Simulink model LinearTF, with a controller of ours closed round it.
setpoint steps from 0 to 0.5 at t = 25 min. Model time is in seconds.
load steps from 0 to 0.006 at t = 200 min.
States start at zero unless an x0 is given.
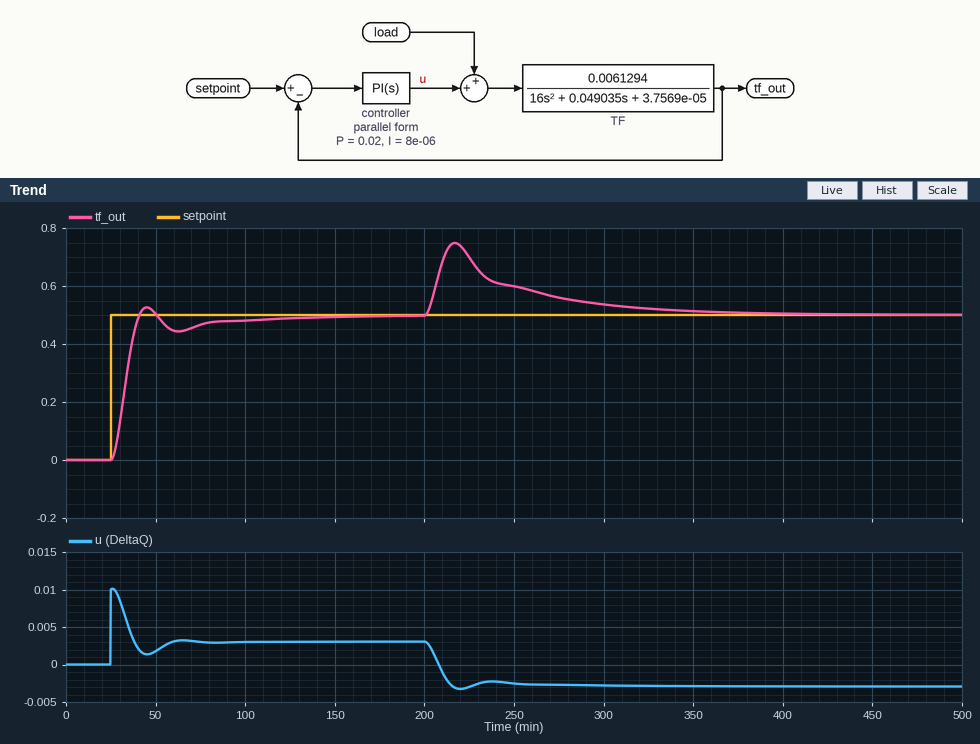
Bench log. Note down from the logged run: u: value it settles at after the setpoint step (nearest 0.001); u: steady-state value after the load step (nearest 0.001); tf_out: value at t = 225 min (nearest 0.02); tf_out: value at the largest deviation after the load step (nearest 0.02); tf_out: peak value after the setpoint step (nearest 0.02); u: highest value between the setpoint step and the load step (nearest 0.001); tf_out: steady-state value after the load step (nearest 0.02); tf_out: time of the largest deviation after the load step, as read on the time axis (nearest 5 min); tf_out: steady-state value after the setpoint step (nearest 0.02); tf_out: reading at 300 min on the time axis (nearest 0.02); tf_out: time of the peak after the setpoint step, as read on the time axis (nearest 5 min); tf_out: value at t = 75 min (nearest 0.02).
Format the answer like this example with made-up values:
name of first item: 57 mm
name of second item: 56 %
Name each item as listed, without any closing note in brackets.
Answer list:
u: value it settles at after the setpoint step: 0.003
u: steady-state value after the load step: -0.003
tf_out: value at t = 225 min: 0.70
tf_out: value at the largest deviation after the load step: 0.74
tf_out: peak value after the setpoint step: 0.52
u: highest value between the setpoint step and the load step: 0.010
tf_out: steady-state value after the load step: 0.50
tf_out: time of the largest deviation after the load step, as read on the time axis: 215 min
tf_out: steady-state value after the setpoint step: 0.50
tf_out: reading at 300 min on the time axis: 0.54
tf_out: time of the peak after the setpoint step, as read on the time axis: 45 min
tf_out: value at t = 75 min: 0.46
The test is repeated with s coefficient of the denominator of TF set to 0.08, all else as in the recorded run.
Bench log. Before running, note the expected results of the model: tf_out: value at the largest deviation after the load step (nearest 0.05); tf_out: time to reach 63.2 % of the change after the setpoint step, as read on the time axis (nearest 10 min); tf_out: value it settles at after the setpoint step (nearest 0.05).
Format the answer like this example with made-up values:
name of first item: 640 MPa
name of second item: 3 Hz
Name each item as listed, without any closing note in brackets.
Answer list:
tf_out: value at the largest deviation after the load step: 0.70
tf_out: time to reach 63.2 % of the change after the setpoint step, as read on the time axis: 40 min
tf_out: value it settles at after the setpoint step: 0.50
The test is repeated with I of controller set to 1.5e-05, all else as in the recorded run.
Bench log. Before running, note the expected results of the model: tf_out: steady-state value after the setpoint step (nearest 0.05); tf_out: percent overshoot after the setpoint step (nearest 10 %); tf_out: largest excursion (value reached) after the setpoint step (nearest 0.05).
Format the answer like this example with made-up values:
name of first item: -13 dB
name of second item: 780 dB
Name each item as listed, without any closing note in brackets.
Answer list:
tf_out: steady-state value after the setpoint step: 0.50
tf_out: percent overshoot after the setpoint step: 20 %
tf_out: largest excursion (value reached) after the setpoint step: 0.60
